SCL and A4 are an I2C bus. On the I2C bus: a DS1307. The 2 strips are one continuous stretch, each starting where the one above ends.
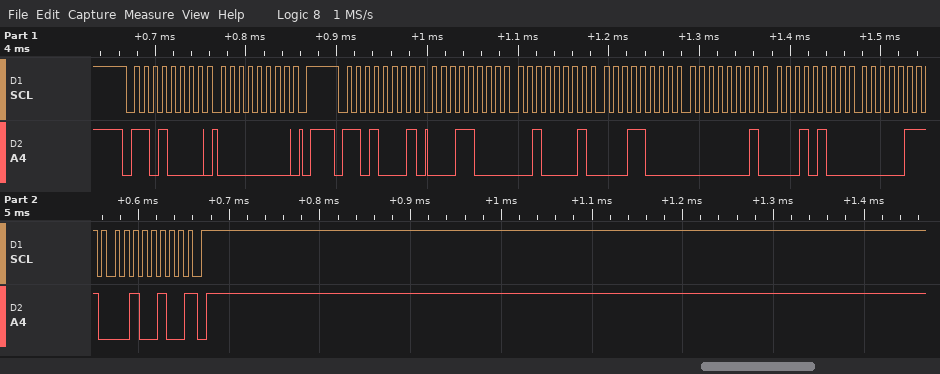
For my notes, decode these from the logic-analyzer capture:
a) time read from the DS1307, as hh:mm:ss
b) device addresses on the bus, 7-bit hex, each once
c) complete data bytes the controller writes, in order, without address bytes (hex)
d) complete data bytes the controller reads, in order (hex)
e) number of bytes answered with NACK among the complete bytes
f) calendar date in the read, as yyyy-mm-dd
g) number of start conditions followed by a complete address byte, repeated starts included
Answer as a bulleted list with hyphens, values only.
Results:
- 18:21:18
- 0x68
- 00
- 18 21 18 01 14 07 24
- 1
- 2024-07-14
- 2
